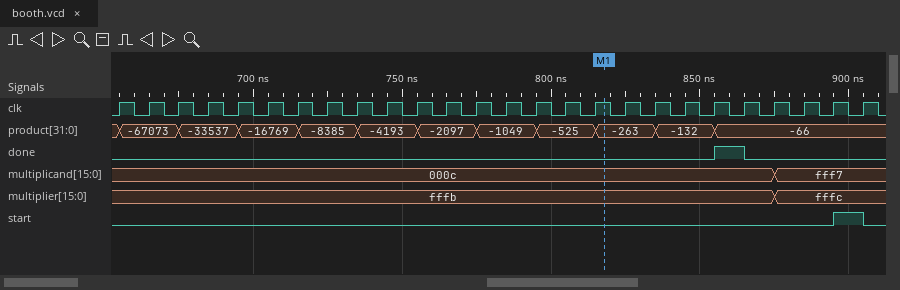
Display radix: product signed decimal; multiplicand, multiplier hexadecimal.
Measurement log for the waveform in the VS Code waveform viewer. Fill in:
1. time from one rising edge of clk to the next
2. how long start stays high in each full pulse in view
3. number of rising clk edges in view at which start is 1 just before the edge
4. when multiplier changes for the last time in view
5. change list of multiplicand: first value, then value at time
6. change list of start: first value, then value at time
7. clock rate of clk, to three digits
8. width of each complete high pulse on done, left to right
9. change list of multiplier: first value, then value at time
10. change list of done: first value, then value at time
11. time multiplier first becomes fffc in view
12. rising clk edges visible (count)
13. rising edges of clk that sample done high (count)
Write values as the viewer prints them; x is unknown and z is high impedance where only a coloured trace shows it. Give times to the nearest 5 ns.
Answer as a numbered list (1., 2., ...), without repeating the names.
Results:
1. 10 ns
2. 10 ns
3. 1
4. 875 ns
5. 000c, fff7 at 875 ns
6. 0, 1 at 895 ns, 0 at 905 ns
7. 100 MHz
8. 10 ns
9. fffb, fffc at 875 ns
10. 0, 1 at 855 ns, 0 at 865 ns
11. 875 ns
12. 26
13. 1
